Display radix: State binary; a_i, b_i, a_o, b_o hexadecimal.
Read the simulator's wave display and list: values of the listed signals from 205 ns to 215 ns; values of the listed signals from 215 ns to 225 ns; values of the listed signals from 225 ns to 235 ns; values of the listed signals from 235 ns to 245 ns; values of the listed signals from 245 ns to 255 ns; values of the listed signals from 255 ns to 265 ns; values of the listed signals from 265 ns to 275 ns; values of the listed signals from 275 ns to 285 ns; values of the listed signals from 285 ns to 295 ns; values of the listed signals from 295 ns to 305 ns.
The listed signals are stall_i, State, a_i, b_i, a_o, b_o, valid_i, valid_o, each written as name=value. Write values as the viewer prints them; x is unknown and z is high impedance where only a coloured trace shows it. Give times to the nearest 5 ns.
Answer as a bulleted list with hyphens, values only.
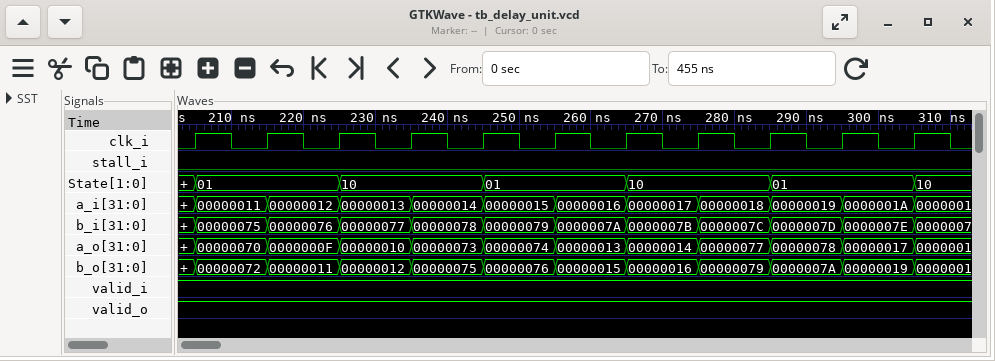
- stall_i=0, State=01, a_i=00000011, b_i=00000075, a_o=00000070, b_o=00000072, valid_i=1, valid_o=1
- stall_i=0, State=01, a_i=00000012, b_i=00000076, a_o=0000000F, b_o=00000011, valid_i=1, valid_o=1
- stall_i=0, State=10, a_i=00000013, b_i=00000077, a_o=00000010, b_o=00000012, valid_i=1, valid_o=1
- stall_i=0, State=10, a_i=00000014, b_i=00000078, a_o=00000073, b_o=00000075, valid_i=1, valid_o=1
- stall_i=0, State=01, a_i=00000015, b_i=00000079, a_o=00000074, b_o=00000076, valid_i=1, valid_o=1
- stall_i=0, State=01, a_i=00000016, b_i=0000007A, a_o=00000013, b_o=00000015, valid_i=1, valid_o=1
- stall_i=0, State=10, a_i=00000017, b_i=0000007B, a_o=00000014, b_o=00000016, valid_i=1, valid_o=1
- stall_i=0, State=10, a_i=00000018, b_i=0000007C, a_o=00000077, b_o=00000079, valid_i=1, valid_o=1
- stall_i=0, State=01, a_i=00000019, b_i=0000007D, a_o=00000078, b_o=0000007A, valid_i=1, valid_o=1
- stall_i=0, State=01, a_i=0000001A, b_i=0000007E, a_o=00000017, b_o=00000019, valid_i=1, valid_o=1
